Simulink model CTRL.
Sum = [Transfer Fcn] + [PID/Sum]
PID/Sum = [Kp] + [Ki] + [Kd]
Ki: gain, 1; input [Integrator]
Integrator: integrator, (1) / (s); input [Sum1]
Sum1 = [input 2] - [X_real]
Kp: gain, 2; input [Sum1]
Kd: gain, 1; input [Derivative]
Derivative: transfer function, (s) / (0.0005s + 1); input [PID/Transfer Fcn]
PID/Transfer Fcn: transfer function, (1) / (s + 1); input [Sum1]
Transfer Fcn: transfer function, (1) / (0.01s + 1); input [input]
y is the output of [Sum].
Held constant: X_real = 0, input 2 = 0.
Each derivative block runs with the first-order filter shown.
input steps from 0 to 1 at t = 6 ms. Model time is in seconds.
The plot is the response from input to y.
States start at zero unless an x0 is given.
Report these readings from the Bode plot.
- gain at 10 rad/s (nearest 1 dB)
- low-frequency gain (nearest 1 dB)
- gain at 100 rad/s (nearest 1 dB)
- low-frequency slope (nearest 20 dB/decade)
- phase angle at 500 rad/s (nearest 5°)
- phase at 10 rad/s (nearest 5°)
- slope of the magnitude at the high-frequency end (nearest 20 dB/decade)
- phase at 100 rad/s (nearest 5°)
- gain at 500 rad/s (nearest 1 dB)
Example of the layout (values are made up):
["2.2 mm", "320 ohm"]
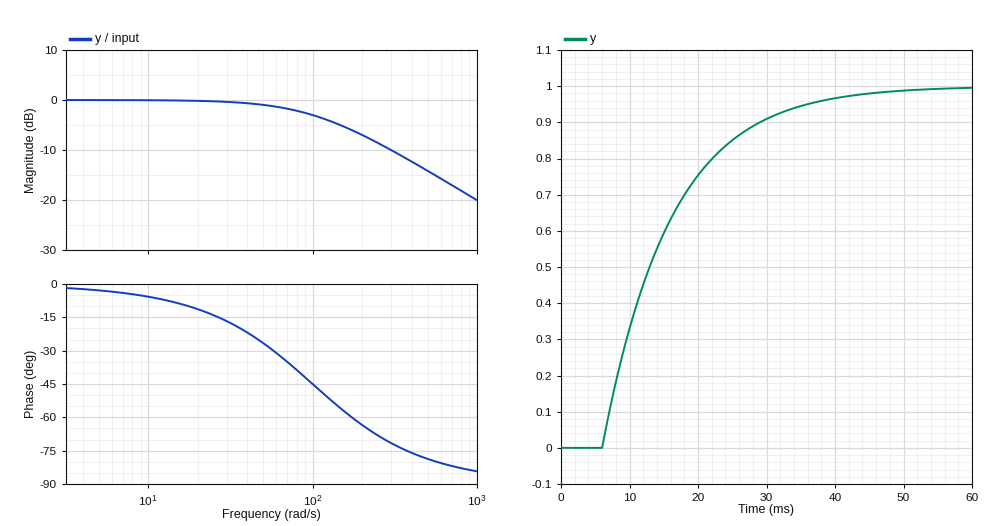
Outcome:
["0 dB", "0 dB", "-3 dB", "0 dB/decade", "-80°", "-5°", "-20 dB/decade", "-45°", "-14 dB"]
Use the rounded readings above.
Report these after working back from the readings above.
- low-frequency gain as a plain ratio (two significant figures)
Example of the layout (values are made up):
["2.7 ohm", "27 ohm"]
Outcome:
["1.0"]
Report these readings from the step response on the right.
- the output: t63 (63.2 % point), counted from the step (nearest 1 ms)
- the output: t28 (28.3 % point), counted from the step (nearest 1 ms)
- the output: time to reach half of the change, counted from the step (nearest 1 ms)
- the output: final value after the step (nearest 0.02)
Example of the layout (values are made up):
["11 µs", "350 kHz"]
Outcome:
["10 ms", "3 ms", "7 ms", "1.00"]
